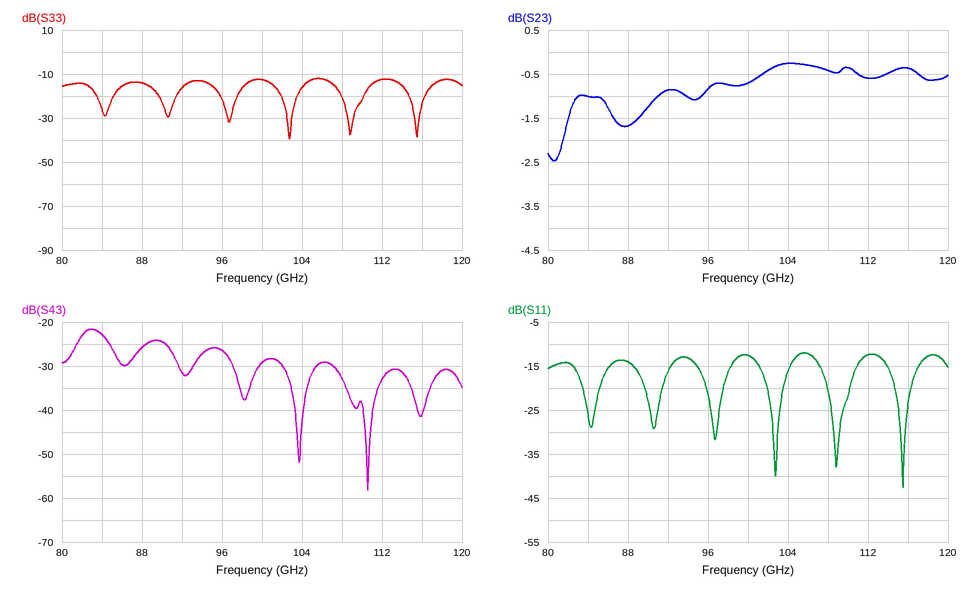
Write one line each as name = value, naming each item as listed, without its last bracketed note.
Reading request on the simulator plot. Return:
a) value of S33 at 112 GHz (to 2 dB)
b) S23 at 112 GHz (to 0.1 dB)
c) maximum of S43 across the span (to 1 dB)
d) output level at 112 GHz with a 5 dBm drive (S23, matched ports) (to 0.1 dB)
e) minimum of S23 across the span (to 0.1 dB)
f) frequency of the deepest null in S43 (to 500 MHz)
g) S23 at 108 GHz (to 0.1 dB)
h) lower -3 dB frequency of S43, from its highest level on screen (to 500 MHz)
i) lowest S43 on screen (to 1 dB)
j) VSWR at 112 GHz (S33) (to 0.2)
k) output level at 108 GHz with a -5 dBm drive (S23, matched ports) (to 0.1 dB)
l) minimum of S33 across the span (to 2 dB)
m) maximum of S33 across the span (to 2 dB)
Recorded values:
value of S33 at 112 GHz = -12 dB
S23 at 112 GHz = -0.6 dB
maximum of S43 across the span = -22 dB
output level at 112 GHz with a 5 dBm drive (S23, matched ports) = 4.4 dBm
minimum of S23 across the span = -2.5 dB
frequency of the deepest null in S43 = 110.5 GHz
S23 at 108 GHz = -0.4 dB
lower -3 dB frequency of S43, from its highest level on screen = 81.5 GHz
lowest S43 on screen = -58 dB
VSWR at 112 GHz (S33) = 1.6
output level at 108 GHz with a -5 dBm drive (S23, matched ports) = -5.4 dBm
minimum of S33 across the span = -40 dB
maximum of S33 across the span = -12 dB
